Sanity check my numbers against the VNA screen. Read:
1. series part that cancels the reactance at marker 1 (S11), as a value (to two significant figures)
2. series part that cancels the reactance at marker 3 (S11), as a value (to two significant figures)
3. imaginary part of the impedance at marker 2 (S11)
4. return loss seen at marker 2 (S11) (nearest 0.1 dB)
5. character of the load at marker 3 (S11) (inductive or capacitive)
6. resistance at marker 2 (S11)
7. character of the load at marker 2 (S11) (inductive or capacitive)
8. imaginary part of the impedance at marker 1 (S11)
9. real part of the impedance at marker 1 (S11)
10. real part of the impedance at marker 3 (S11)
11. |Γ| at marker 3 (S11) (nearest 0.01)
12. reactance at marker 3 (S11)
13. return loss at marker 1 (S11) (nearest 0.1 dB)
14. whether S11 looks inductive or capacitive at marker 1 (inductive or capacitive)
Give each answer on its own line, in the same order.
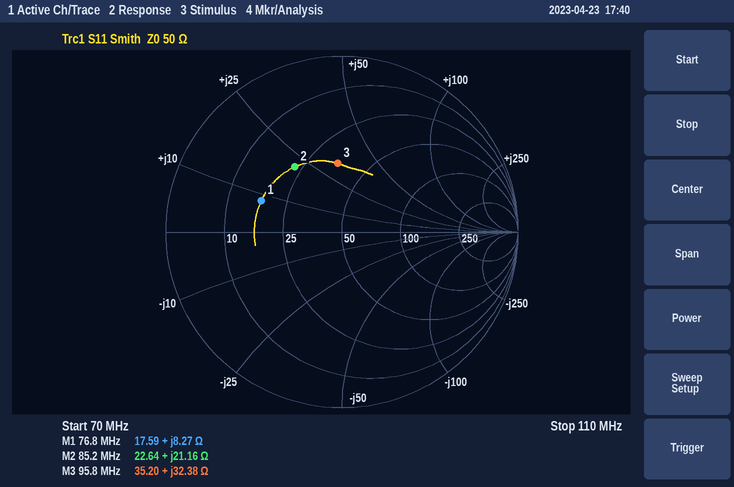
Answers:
250 pF
51 pF
+21.16 Ω
6.8 dB
inductive
22.64 Ω
inductive
+8.27 Ω
17.59 Ω
35.20 Ω
0.39
+32.38 Ω
6.2 dB
inductive
